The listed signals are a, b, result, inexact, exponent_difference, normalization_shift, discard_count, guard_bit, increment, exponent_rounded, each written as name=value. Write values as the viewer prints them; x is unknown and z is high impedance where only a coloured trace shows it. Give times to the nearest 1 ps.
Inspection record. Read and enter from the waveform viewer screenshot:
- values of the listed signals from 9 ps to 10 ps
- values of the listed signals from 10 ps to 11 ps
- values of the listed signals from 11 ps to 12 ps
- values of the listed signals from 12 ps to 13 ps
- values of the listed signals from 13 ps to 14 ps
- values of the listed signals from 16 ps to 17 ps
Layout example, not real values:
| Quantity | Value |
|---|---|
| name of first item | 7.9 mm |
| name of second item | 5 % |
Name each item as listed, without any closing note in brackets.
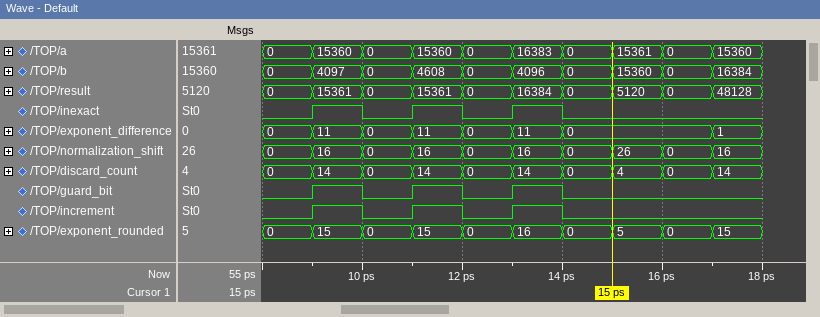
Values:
| Quantity | Value |
|---|---|
| values of the listed signals from 9 ps to 10 ps | a=15360, b=4097, result=15361, inexact=1, exponent_difference=11, normalization_shift=16, discard_count=14, guard_bit=1, increment=1, exponent_rounded=15 |
| values of the listed signals from 10 ps to 11 ps | a=0, b=0, result=0, inexact=0, exponent_difference=0, normalization_shift=0, discard_count=0, guard_bit=0, increment=0, exponent_rounded=0 |
| values of the listed signals from 11 ps to 12 ps | a=15360, b=4608, result=15361, inexact=1, exponent_difference=11, normalization_shift=16, discard_count=14, guard_bit=1, increment=1, exponent_rounded=15 |
| values of the listed signals from 12 ps to 13 ps | a=0, b=0, result=0, inexact=0, exponent_difference=0, normalization_shift=0, discard_count=0, guard_bit=0, increment=0, exponent_rounded=0 |
| values of the listed signals from 13 ps to 14 ps | a=16383, b=4096, result=16384, inexact=1, exponent_difference=11, normalization_shift=16, discard_count=14, guard_bit=1, increment=1, exponent_rounded=16 |
| values of the listed signals from 16 ps to 17 ps | a=0, b=0, result=0, inexact=0, exponent_difference=0, normalization_shift=0, discard_count=0, guard_bit=0, increment=0, exponent_rounded=0 |
